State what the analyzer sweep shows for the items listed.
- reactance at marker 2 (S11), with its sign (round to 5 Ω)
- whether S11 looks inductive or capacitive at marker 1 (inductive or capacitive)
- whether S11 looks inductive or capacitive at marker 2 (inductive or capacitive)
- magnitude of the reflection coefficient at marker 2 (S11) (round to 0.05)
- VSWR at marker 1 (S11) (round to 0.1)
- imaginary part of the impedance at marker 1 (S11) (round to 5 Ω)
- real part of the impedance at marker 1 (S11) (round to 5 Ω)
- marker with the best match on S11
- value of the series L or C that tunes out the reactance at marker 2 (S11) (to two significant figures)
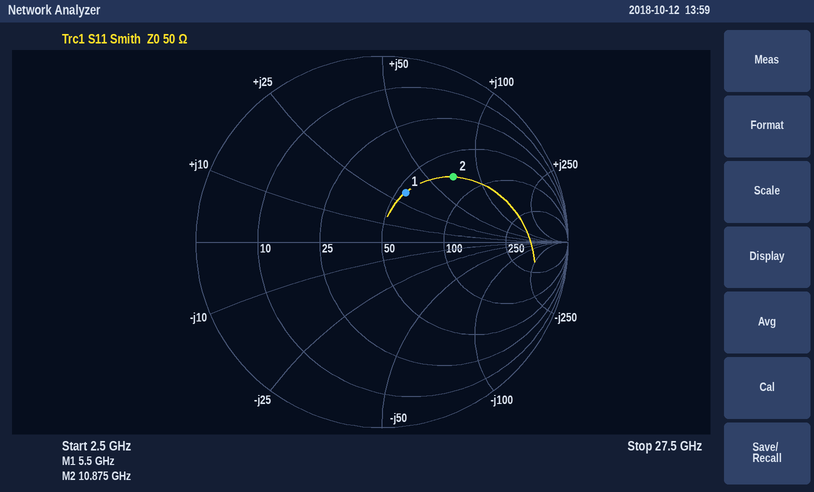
+70 Ω
inductive
inductive
0.50
1.8
+30 Ω
55 Ω
marker 1
210 fF
